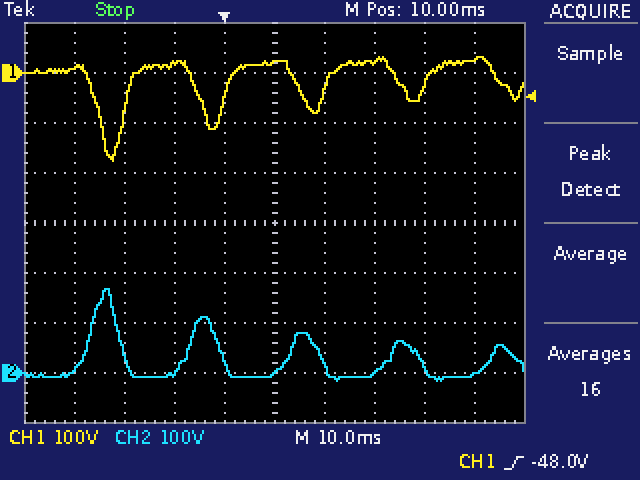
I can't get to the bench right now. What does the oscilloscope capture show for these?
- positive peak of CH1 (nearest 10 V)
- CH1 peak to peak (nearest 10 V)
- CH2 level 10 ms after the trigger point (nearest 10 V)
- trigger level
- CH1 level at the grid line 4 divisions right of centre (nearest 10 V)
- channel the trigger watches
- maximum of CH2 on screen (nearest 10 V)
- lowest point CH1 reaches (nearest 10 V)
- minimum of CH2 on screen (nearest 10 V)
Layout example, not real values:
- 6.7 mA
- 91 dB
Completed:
- 30 V
- 210 V
- 0 V
- -48.0 V
- 30 V
- CH1
- 170 V
- -180 V
- -20 V
